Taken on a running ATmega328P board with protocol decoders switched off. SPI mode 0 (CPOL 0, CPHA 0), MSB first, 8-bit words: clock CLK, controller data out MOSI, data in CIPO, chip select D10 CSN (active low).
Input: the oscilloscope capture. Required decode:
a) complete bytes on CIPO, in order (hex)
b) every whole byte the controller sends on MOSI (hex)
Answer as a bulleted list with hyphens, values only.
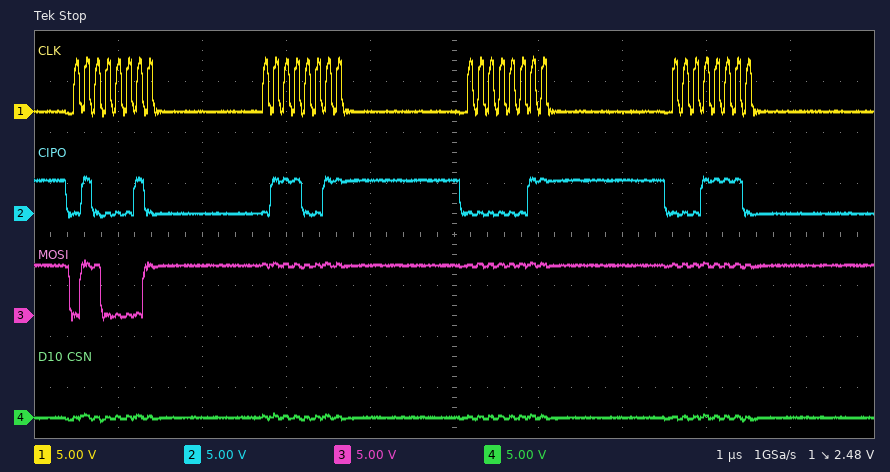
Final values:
- 0x42 0x73 0x03 0x1E
- 0x61 0xFF 0xFF 0xFF
